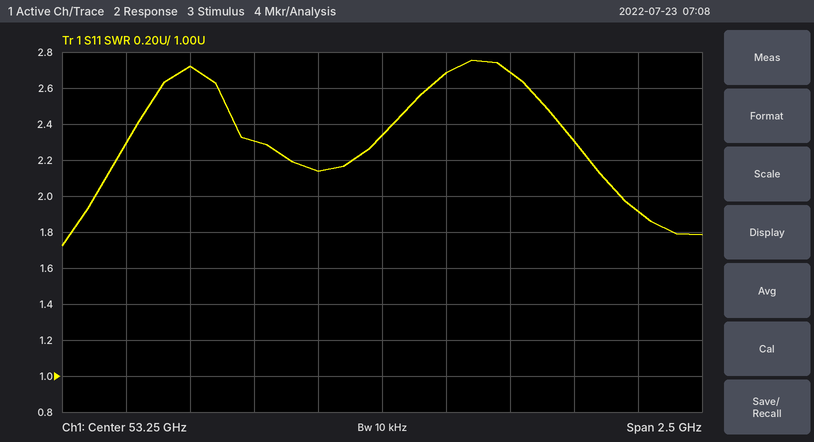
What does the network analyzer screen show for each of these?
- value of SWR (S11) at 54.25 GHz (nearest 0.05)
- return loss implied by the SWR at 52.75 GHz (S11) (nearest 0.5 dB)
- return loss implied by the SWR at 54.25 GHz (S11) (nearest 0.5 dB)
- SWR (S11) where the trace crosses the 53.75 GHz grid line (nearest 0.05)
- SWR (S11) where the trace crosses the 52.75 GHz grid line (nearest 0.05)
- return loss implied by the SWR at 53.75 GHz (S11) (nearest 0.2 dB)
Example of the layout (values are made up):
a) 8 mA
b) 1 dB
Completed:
a) 1.90
b) 8.0 dB
c) 10.0 dB
d) 2.70
e) 2.30
f) 6.8 dB
